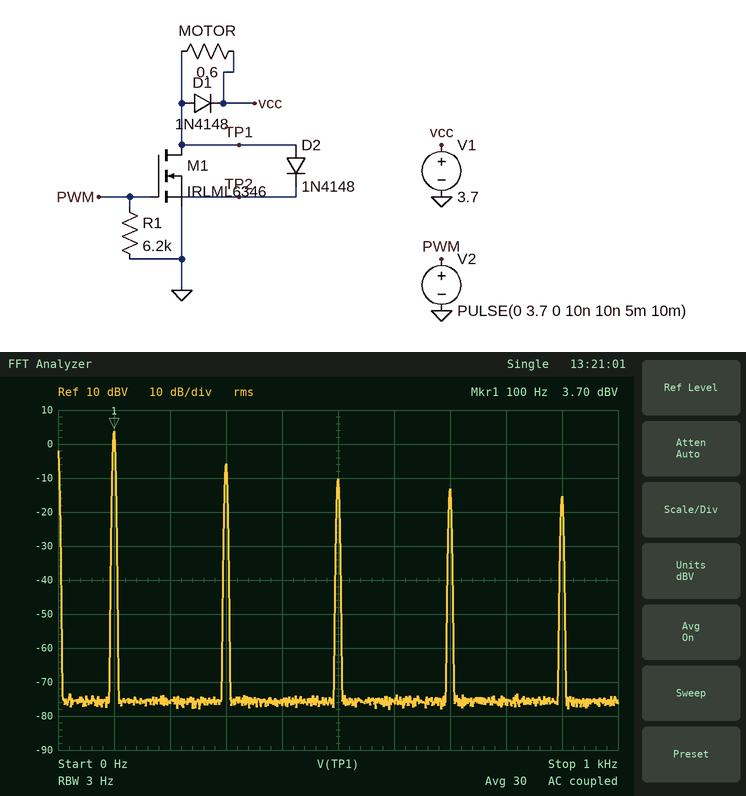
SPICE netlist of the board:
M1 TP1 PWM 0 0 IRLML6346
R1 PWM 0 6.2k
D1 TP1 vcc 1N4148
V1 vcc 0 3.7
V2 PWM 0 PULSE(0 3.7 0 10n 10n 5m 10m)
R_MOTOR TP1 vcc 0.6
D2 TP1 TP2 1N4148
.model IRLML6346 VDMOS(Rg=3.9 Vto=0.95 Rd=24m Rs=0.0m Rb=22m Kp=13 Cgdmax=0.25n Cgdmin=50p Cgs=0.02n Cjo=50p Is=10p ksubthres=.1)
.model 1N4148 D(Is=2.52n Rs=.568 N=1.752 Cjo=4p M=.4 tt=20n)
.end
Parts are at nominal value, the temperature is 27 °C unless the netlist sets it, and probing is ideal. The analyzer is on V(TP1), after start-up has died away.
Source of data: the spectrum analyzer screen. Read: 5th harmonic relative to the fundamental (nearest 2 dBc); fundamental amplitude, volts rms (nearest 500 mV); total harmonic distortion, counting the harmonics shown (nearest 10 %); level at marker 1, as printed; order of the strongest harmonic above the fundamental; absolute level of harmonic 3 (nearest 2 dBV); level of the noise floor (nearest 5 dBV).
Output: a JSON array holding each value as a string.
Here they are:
["-14 dBc", "1.5 V", "40 %", "3.70 dBV", "3", "-6 dBV", "-75 dBV"]
